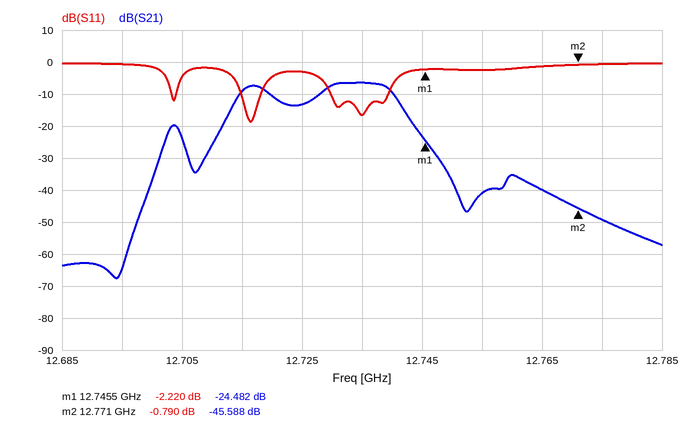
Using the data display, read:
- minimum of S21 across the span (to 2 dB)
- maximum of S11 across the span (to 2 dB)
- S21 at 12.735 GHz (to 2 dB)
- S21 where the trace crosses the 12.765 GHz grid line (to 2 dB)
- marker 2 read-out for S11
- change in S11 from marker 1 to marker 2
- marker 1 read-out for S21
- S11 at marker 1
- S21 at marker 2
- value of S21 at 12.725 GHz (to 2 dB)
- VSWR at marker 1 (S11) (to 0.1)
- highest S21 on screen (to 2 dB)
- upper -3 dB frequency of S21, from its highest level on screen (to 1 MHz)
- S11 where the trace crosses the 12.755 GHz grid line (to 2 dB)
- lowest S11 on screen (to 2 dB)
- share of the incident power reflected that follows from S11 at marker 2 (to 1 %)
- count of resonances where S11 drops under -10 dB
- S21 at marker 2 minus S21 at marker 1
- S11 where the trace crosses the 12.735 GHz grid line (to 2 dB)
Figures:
-68 dB
0 dB
-6 dB
-40 dB
-0.790 dB
1.430 dB
-24.482 dB
-2.220 dB
-45.588 dB
-14 dB
7.9
-6 dB
12.740 GHz
-2 dB
-18 dB
83 %
3
-21.106 dB
-16 dB
